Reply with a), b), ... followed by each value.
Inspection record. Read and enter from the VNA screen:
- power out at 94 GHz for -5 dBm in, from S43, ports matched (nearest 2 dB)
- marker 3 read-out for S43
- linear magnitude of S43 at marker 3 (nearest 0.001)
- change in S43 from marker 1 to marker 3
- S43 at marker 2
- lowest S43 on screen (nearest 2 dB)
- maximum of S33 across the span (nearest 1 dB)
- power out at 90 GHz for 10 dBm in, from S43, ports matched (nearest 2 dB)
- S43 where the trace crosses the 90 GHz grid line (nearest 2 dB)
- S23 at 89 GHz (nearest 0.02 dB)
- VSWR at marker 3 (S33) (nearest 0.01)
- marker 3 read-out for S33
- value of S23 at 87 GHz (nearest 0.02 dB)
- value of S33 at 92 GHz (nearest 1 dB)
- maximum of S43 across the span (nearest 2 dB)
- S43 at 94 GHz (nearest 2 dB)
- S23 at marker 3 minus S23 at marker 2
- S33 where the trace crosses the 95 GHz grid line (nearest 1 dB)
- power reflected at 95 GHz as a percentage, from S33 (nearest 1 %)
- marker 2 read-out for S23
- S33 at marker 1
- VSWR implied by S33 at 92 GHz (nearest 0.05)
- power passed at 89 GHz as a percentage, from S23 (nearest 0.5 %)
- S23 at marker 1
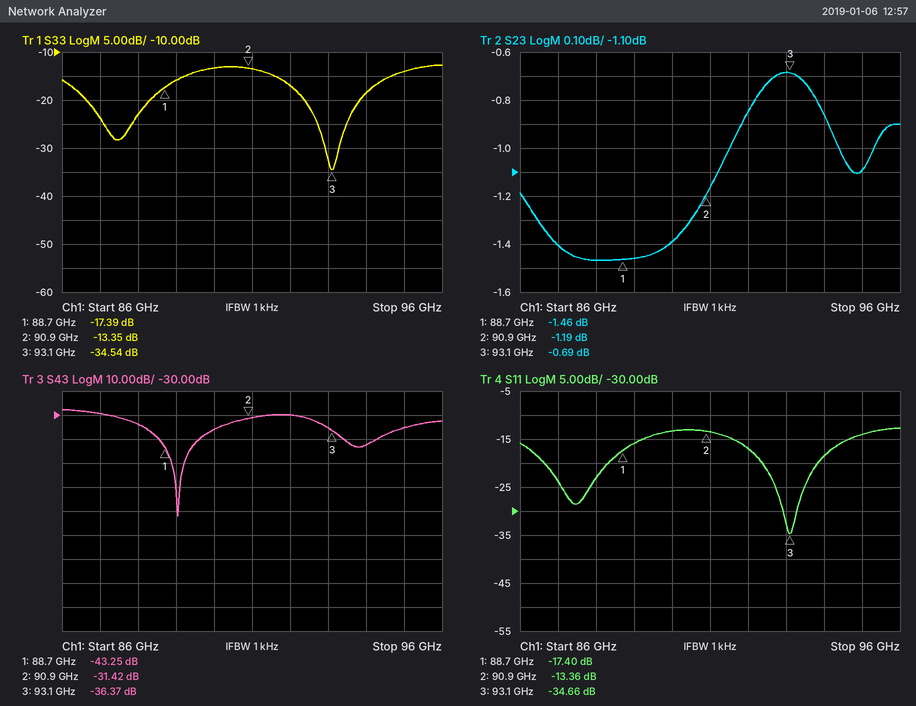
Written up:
a) -48 dBm
b) -36.37 dB
c) 0.015
d) 6.88 dB
e) -31.42 dB
f) -72 dB
g) -13 dB
h) -26 dBm
i) -36 dB
j) -1.46 dB
k) 1.04
l) -34.54 dB
m) -1.40 dB
n) -17 dB
o) -28 dB
p) -42 dB
q) 0.50 dB
r) -14 dB
s) 4 %
t) -1.19 dB
u) -17.39 dB
v) 1.35
w) 71.5 %
x) -1.46 dB
